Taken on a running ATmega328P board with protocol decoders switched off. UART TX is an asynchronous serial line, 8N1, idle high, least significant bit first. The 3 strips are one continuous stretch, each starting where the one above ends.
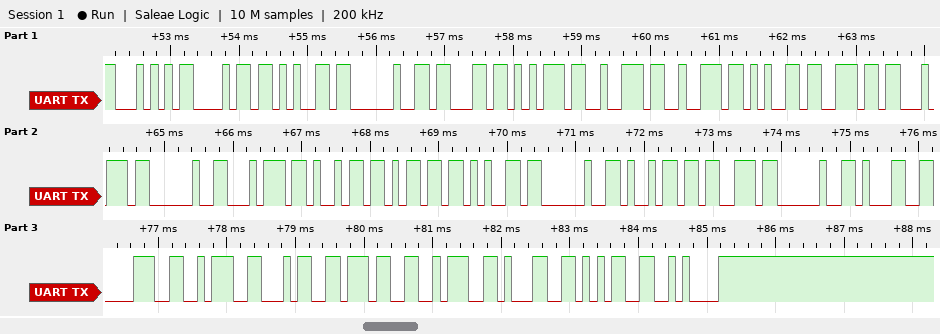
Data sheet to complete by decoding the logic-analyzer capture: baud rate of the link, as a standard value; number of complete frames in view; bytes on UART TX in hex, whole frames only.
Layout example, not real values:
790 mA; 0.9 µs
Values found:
9600 baud; 29; 54 68 65 20 63 75 72 72 65 6E 74 20 74 69 6D 65 20 69 73 20 31 38 3A 34 37 3A 31 35 0A
